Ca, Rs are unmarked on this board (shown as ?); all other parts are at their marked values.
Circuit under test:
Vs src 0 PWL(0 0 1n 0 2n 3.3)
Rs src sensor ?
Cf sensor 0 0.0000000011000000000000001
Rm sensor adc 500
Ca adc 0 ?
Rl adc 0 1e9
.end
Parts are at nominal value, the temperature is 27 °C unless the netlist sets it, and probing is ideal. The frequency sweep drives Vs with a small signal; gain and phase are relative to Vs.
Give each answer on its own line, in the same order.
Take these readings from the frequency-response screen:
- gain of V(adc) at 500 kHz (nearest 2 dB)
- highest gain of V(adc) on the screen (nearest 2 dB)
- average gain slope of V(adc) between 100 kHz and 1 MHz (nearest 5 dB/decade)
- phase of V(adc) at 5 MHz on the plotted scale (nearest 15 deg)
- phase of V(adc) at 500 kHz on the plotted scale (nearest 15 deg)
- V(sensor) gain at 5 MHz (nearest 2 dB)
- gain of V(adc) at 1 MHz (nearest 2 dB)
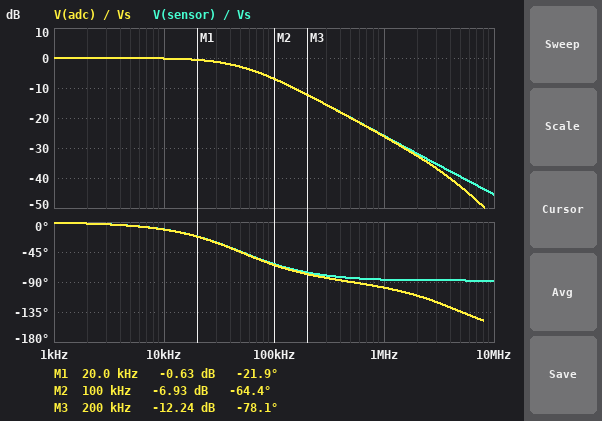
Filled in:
-20 dB
0 dB
-20 dB/decade
-135 deg
-90 deg
-40 dB
-26 dB
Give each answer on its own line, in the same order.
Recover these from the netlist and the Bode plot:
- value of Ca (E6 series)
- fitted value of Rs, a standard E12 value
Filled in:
68 pF
2.7 kΩ
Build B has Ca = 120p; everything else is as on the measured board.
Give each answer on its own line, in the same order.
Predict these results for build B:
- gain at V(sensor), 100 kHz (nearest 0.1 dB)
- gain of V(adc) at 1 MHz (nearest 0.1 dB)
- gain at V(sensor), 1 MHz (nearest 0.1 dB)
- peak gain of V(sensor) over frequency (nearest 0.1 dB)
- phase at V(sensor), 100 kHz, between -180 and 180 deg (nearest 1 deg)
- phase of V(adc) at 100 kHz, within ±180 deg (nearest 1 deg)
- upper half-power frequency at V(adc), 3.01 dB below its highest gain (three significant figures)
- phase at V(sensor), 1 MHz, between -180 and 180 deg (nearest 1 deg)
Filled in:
-7.2 dB
-26.8 dB
-26.2 dB
0 dB
-64 deg
-66 deg
48.2 kHz
-85 deg
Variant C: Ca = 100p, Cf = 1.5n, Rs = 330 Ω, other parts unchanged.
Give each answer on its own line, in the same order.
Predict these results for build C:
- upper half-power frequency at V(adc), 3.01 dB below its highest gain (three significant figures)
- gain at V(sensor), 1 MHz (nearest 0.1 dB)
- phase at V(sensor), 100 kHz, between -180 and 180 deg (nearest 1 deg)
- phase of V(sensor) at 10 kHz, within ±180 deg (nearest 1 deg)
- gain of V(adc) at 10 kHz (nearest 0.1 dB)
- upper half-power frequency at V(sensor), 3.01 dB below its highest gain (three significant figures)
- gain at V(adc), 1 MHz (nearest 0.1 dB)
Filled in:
297 kHz
-10.8 dB
-18 deg
-2 deg
0 dB
300 kHz
-11.2 dB
